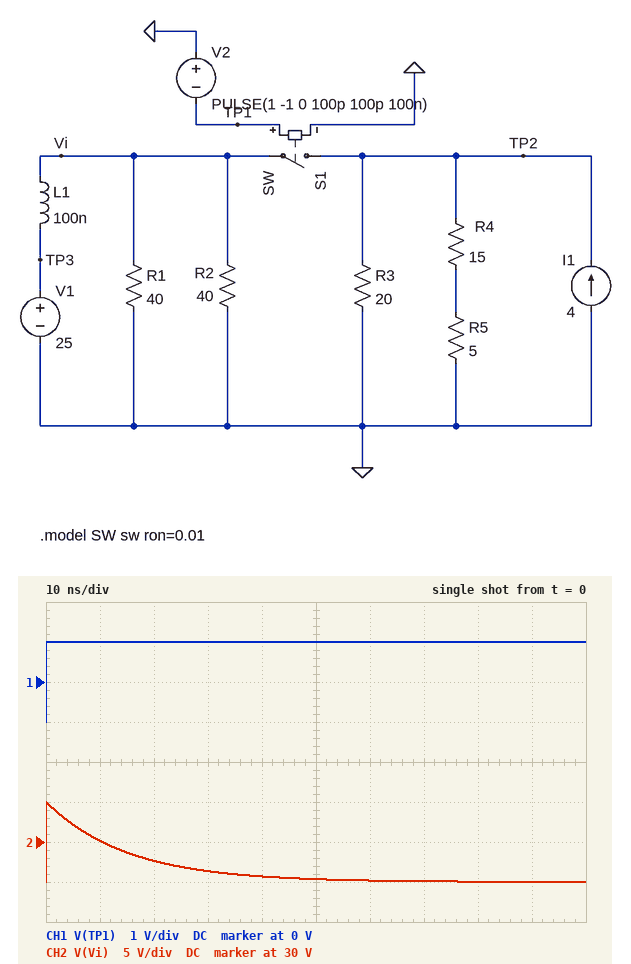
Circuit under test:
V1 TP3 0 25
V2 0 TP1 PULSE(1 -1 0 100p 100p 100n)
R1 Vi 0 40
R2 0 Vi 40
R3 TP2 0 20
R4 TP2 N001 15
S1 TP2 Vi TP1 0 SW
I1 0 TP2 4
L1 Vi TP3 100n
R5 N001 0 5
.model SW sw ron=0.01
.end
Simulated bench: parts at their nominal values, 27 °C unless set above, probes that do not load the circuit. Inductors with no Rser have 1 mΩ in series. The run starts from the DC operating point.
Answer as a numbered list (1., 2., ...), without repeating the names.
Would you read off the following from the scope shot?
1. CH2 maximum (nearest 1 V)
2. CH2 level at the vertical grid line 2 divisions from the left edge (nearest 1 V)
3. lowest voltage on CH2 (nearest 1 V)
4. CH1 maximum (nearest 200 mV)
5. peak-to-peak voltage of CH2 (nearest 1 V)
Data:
1. 35 V
2. 28 V
3. 25 V
4. 1.0 V
5. 10 V
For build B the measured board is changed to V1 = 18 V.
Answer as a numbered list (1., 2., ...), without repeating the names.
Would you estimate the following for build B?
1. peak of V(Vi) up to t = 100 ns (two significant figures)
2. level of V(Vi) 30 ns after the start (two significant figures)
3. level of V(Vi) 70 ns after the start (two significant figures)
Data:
1. 33 V
2. 20 V
3. 18 V
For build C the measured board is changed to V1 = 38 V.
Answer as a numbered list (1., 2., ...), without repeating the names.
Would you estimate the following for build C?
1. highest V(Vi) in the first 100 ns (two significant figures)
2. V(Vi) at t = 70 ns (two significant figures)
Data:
1. 39 V
2. 38 V
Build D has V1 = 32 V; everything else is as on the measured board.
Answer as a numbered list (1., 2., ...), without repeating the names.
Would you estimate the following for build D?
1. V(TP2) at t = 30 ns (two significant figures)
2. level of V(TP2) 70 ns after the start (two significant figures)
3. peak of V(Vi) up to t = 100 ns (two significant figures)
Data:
1. 33 V
2. 32 V
3. 37 V
